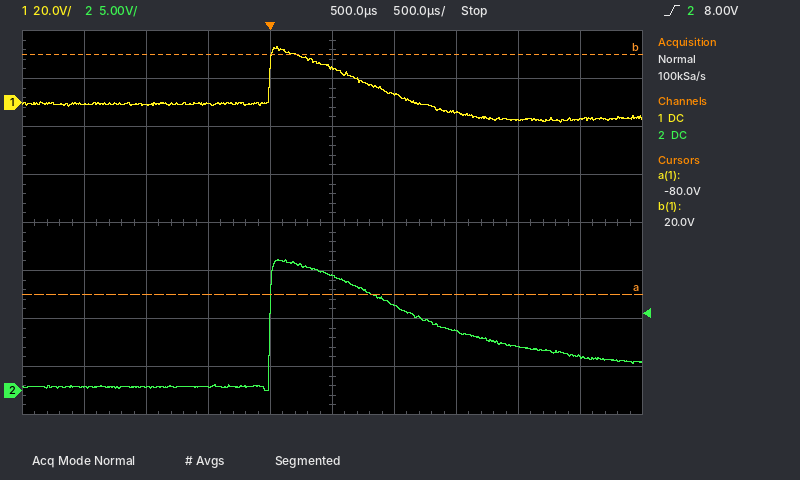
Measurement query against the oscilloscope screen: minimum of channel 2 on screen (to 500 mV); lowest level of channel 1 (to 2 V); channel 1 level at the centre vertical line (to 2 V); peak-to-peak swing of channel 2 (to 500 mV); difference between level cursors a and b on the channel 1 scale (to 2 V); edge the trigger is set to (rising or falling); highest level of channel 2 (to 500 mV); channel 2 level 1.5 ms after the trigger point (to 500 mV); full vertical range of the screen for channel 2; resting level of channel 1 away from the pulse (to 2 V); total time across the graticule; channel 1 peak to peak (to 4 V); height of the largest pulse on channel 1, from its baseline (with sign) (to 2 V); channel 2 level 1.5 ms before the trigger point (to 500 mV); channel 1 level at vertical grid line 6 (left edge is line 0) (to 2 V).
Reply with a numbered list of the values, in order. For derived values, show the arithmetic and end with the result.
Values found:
1. 0.0 V
2. -8 V
3. 14 V
4. 13.5 V − (0.0 V) = 13.5 V
5. 100 V
6. rising
7. 13.5 V
8. 6.0 V
9. 40 V
10. 0 V
11. 5 ms
12. 32 V
13. +24 V
14. 500 mV
15. 4 V
